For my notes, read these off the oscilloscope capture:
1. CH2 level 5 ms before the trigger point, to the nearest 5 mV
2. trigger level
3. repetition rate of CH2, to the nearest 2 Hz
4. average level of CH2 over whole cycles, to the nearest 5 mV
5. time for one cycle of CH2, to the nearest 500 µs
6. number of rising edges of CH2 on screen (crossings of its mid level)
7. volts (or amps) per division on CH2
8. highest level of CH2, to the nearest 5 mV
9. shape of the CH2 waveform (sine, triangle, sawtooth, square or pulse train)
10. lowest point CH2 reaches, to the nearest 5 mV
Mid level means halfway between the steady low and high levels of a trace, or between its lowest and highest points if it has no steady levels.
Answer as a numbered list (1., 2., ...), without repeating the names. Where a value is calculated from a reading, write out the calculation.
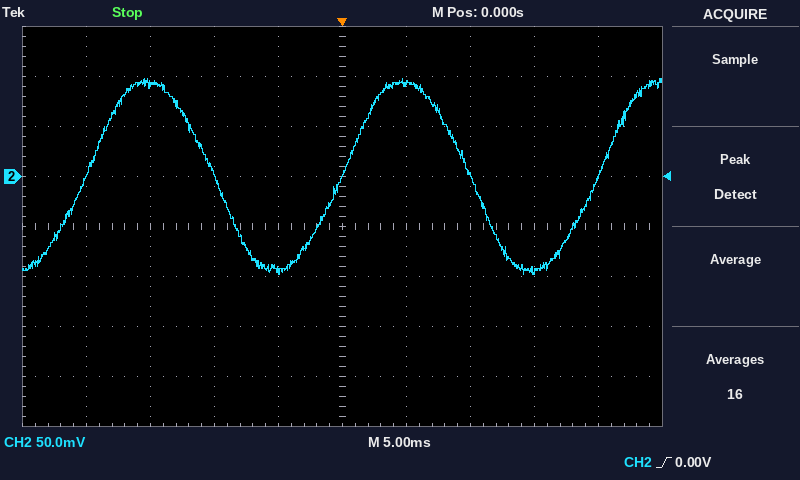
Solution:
1. -95 mV
2. 0.00 V
3. 1 / 20.0 ms ≈ 50 Hz
4. (100 mV + (-100 mV)) / 2 ≈ 0 mV
5. 20.0 ms
6. 3
7. 50 mV
8. 100 mV
9. sine
10. -100 mV
